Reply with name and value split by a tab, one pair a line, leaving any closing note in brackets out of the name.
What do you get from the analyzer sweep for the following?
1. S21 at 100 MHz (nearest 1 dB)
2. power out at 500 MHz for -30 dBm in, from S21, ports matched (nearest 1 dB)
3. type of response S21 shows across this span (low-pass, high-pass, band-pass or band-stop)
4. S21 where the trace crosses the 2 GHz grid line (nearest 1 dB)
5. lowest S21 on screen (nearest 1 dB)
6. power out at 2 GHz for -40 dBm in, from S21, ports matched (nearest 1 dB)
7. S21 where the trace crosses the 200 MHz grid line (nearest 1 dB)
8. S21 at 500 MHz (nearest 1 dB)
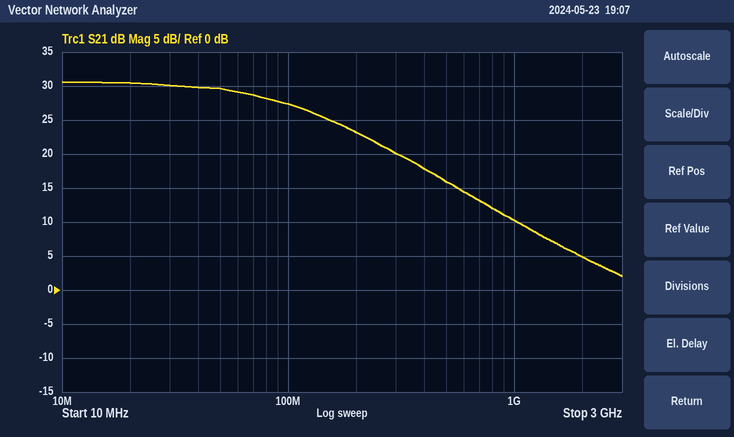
S21 at 100 MHz	27 dB
power out at 500 MHz for -30 dBm in, from S21, ports matched	-14 dBm
type of response S21 shows across this span	low-pass
S21 where the trace crosses the 2 GHz grid line	5 dB
lowest S21 on screen	2 dB
power out at 2 GHz for -40 dBm in, from S21, ports matched	-35 dBm
S21 where the trace crosses the 200 MHz grid line	23 dB
S21 at 500 MHz	16 dB
